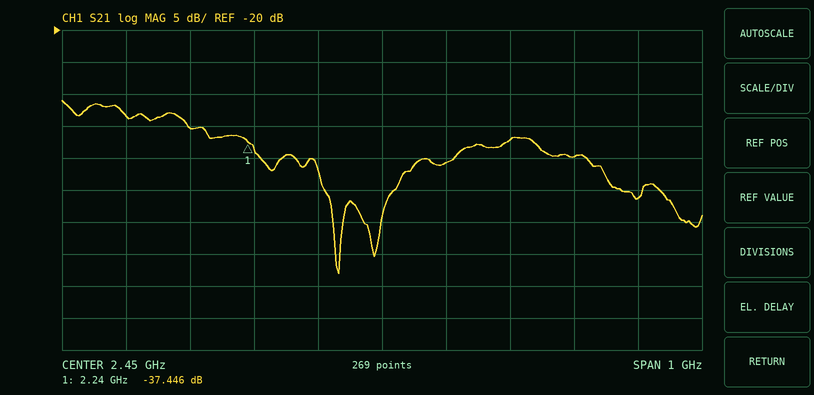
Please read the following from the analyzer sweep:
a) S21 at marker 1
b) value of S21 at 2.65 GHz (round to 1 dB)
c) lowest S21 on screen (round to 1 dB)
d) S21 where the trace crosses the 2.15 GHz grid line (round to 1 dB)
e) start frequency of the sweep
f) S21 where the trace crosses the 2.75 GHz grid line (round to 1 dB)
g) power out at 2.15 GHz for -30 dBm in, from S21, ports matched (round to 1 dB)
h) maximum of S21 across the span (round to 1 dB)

-37.446 dB
-37 dB
-58 dB
-35 dB
1.95 GHz
-40 dB
-65 dBm
-31 dB
